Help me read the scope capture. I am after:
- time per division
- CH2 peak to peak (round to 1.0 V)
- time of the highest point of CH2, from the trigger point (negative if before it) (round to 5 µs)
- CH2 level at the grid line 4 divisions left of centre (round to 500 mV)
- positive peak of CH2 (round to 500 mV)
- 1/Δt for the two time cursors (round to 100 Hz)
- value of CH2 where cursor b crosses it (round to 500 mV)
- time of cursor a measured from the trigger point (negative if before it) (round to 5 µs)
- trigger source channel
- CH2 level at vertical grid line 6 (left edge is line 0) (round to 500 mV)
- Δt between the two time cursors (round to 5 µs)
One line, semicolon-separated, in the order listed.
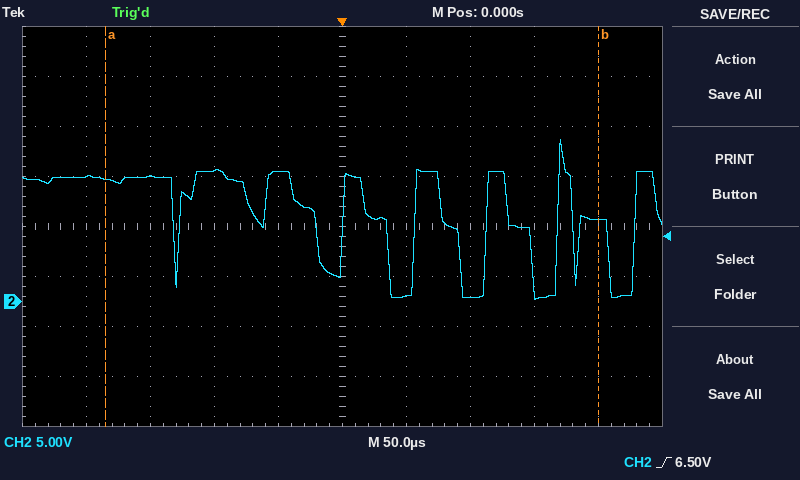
50 µs; 16.0 V; +170 µs; 12.5 V; 16.0 V; 2.6 kHz; 8.0 V; -185 µs; CH2; 500 mV; 385 µs
